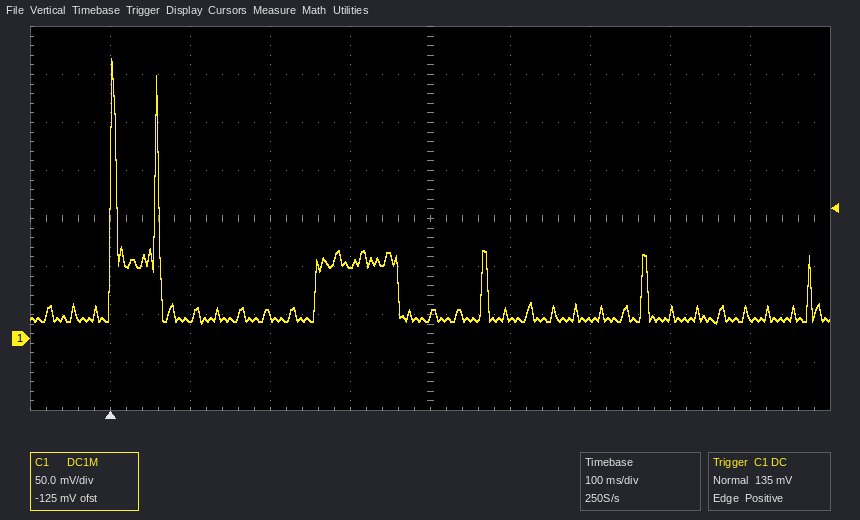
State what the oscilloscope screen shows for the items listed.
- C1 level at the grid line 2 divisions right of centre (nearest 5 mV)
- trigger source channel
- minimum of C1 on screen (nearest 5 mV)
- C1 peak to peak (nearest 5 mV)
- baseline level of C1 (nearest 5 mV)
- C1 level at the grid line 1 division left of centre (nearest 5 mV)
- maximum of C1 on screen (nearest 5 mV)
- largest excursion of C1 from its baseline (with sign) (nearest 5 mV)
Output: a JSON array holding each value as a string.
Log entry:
["20 mV", "C1", "15 mV", "275 mV", "20 mV", "75 mV", "290 mV", "+270 mV"]
